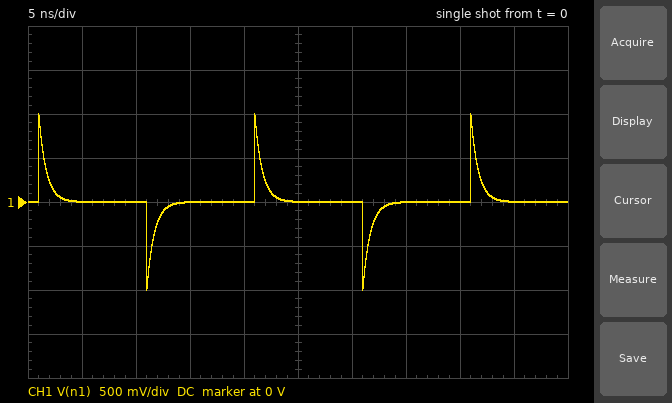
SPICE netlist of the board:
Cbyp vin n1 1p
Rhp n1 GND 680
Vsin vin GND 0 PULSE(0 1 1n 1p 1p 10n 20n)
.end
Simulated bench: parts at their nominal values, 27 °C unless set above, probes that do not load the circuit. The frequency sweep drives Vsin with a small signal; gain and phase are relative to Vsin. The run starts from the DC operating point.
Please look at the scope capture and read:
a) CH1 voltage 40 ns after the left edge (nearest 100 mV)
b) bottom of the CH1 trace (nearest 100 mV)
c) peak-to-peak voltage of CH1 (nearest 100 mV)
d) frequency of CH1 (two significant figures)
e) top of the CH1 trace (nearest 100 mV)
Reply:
0 V
-1.0 V
2.0 V
50 MHz
1.0 V
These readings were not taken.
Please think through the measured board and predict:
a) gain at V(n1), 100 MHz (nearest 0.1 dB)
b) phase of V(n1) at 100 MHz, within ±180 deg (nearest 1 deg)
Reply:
-8.1 dB
67 deg
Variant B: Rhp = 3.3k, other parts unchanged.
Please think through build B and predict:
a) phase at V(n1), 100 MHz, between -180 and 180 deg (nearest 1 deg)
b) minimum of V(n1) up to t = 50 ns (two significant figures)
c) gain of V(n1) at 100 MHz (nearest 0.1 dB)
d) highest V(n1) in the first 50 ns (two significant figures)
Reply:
26 deg
-950 mV
-0.9 dB
1.0 V
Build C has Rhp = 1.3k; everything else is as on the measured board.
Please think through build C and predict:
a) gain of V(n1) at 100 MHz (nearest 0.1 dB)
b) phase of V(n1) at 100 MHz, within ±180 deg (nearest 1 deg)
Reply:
-4.0 dB
51 deg
